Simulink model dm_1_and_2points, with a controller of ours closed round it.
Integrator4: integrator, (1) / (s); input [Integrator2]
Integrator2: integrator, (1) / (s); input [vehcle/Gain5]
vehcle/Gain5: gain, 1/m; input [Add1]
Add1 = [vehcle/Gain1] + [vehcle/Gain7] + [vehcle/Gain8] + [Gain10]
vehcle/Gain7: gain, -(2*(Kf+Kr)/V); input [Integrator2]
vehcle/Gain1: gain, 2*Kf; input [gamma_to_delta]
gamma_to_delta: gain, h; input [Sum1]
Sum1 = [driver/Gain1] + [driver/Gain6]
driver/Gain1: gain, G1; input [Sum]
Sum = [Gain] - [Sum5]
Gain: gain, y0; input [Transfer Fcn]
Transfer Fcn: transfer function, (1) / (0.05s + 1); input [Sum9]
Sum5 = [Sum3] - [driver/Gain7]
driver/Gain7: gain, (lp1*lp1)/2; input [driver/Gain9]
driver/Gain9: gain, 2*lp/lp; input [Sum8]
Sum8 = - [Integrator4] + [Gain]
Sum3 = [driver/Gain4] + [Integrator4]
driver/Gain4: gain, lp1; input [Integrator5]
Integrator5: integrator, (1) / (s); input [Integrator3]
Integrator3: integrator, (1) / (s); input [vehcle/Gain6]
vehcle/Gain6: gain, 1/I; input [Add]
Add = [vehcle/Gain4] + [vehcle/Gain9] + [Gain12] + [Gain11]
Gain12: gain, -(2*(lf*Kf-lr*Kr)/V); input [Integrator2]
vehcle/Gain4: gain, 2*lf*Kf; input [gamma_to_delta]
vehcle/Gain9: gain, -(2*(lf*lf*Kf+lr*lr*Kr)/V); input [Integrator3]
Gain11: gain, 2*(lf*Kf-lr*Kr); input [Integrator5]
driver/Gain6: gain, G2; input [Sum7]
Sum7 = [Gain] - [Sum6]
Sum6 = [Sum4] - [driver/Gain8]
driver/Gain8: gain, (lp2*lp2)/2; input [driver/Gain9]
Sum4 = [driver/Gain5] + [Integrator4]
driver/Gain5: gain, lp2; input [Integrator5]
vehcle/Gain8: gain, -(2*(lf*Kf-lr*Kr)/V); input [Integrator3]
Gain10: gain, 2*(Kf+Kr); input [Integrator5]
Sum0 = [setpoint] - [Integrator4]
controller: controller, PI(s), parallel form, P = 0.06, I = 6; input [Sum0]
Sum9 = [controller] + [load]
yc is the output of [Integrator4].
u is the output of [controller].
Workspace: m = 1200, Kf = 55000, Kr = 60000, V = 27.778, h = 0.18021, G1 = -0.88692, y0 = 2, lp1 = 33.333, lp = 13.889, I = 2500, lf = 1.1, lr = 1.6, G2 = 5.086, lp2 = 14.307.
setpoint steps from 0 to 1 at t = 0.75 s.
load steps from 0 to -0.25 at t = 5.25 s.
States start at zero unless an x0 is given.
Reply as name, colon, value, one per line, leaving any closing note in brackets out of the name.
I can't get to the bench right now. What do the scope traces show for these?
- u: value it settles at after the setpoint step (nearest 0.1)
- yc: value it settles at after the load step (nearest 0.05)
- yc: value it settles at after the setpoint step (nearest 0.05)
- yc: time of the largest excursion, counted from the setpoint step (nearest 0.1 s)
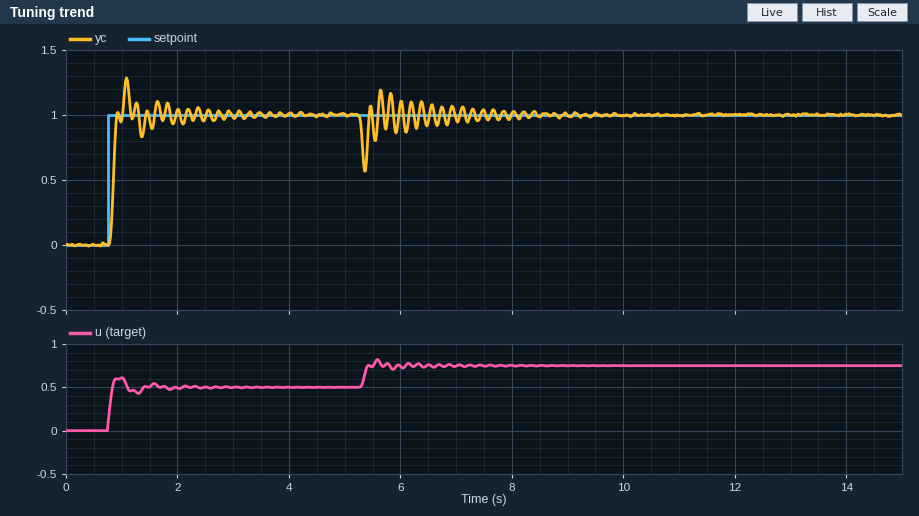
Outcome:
u: value it settles at after the setpoint step: 0.5
yc: value it settles at after the load step: 1.00
yc: value it settles at after the setpoint step: 1.00
yc: time of the largest excursion, counted from the setpoint step: 0.3 s
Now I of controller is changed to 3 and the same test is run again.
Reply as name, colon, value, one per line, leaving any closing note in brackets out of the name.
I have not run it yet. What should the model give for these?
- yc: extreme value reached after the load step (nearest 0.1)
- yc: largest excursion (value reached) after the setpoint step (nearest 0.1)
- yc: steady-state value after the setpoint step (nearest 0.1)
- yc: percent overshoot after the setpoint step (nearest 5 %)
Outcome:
yc: extreme value reached after the load step: 0.5
yc: largest excursion (value reached) after the setpoint step: 1.1
yc: steady-state value after the setpoint step: 1.0
yc: percent overshoot after the setpoint step: 10 %
